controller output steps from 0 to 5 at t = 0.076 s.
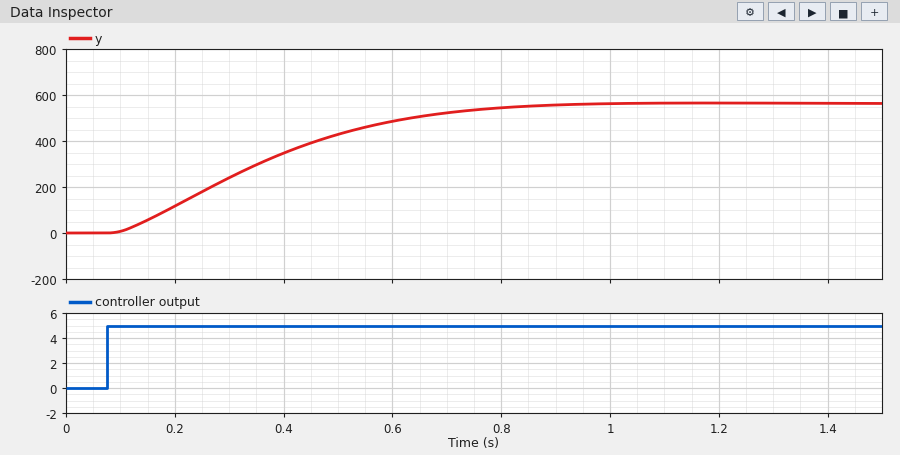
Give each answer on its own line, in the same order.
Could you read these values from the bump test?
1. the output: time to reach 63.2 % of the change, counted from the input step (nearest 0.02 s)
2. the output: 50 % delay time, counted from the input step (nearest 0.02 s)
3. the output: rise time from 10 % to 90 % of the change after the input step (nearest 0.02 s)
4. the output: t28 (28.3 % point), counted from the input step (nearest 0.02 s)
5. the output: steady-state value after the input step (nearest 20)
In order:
0.34 s
0.26 s
0.50 s
0.16 s
560
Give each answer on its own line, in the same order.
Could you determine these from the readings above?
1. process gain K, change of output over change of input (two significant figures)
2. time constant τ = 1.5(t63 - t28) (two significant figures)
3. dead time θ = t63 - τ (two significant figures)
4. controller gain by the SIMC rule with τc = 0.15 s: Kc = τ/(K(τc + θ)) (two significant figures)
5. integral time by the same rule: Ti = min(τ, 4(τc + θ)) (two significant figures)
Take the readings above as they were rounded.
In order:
110
0.27 s
0.070 s
0.011
0.27 s
